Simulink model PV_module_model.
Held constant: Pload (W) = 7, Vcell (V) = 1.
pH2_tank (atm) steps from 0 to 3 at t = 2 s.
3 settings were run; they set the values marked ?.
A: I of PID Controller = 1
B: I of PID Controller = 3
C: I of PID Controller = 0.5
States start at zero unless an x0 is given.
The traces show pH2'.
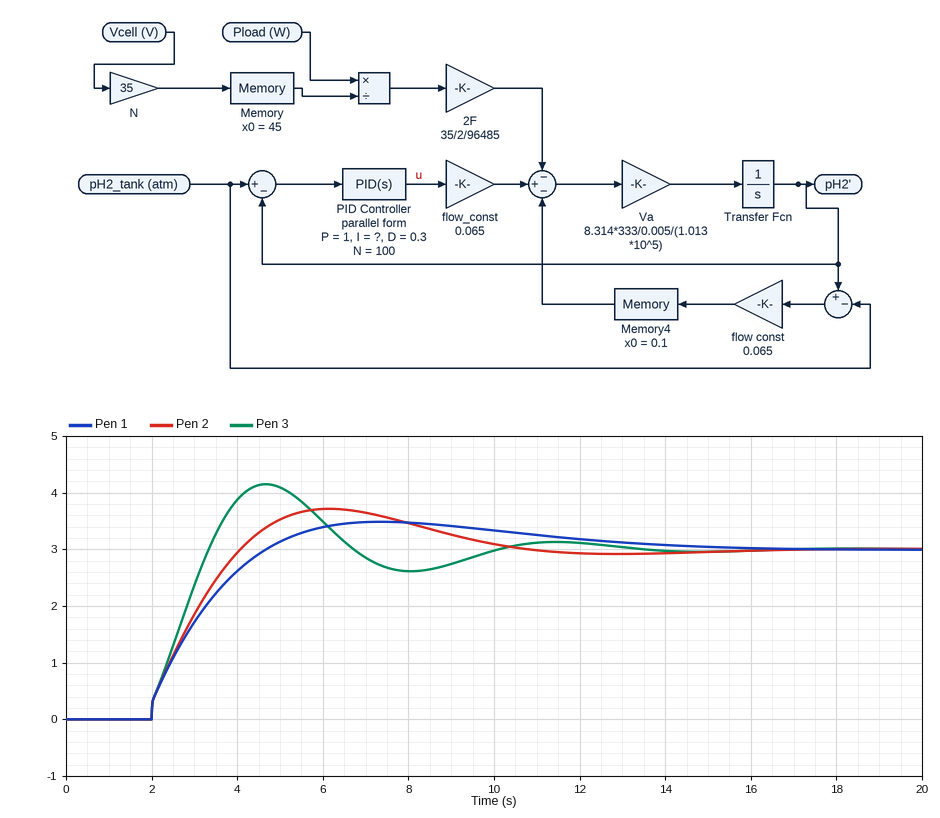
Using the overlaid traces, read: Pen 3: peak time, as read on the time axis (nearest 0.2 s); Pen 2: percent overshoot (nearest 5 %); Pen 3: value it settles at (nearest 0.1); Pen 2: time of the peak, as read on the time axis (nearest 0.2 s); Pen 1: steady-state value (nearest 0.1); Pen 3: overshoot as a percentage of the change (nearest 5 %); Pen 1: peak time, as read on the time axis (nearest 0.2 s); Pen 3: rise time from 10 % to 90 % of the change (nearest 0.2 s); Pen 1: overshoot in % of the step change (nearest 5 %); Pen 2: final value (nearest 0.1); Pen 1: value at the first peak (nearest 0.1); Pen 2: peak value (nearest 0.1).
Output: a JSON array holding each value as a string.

["4.6 s", "25 %", "3.0", "6.2 s", "3.0", "40 %", "7.4 s", "1.2 s", "15 %", "3.0", "3.5", "3.7"]
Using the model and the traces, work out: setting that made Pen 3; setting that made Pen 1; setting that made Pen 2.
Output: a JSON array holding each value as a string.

["B", "C", "A"]
